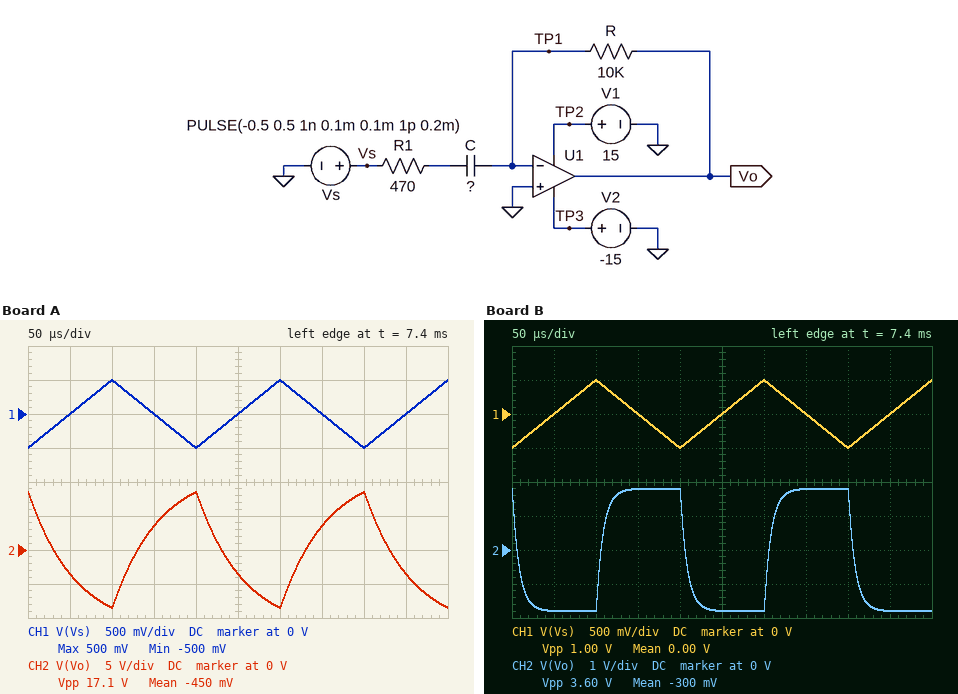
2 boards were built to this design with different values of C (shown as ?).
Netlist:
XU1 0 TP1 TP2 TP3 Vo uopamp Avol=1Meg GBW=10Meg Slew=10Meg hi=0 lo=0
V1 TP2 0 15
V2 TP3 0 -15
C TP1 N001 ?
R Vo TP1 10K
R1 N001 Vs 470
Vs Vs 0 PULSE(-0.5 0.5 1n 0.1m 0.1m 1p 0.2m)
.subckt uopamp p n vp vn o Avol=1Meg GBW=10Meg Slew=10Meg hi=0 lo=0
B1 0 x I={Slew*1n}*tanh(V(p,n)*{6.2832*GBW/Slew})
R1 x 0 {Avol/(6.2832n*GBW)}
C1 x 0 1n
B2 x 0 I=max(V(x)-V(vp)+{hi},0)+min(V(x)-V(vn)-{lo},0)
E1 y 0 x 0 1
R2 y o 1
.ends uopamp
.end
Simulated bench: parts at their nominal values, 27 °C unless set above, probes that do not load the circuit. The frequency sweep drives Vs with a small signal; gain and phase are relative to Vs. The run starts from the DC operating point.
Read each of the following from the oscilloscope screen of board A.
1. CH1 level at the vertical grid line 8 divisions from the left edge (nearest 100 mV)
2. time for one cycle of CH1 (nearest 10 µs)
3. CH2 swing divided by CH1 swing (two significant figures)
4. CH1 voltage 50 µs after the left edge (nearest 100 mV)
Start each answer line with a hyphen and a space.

- -500 mV
- 200 µs
- 17
- 0 V
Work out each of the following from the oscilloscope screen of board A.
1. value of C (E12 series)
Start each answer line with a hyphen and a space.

- 120 nF
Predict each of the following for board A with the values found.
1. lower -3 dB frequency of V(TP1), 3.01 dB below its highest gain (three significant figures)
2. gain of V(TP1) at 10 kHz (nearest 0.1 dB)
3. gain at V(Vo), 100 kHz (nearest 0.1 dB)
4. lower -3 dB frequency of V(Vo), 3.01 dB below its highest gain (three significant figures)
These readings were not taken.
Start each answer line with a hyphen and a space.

- 446 kHz
- -33.7 dB
- 26.4 dB
- 2.80 kHz
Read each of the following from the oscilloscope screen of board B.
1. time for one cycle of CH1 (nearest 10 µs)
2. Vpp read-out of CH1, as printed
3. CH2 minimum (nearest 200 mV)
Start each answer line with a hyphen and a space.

- 200 µs
- 1.00 V
- -1.8 V
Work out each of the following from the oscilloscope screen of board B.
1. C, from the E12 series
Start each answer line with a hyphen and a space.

- 18 nF
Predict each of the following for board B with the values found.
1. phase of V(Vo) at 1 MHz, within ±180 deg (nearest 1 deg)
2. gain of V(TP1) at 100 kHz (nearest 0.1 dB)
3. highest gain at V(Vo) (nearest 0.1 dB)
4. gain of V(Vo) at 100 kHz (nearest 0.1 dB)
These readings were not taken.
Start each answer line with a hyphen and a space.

- 114 deg
- -13.5 dB
- 26.5 dB
- 26.5 dB
